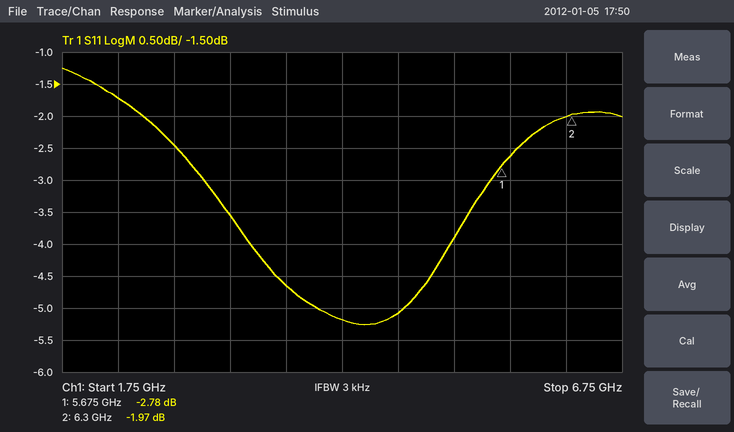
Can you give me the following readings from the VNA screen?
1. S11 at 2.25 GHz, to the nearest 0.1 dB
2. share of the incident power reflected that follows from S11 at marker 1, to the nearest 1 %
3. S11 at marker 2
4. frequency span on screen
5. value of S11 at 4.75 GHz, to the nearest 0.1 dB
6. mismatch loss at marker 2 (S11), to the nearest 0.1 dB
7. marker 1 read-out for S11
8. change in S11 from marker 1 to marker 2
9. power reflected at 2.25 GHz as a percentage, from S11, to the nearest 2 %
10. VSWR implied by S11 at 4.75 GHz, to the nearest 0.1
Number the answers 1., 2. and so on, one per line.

1. -1.7 dB
2. 53 %
3. -1.97 dB
4. 5 GHz
5. -5.1 dB
6. 4.4 dB
7. -2.78 dB
8. 0.81 dB
9. 68 %
10. 3.5
